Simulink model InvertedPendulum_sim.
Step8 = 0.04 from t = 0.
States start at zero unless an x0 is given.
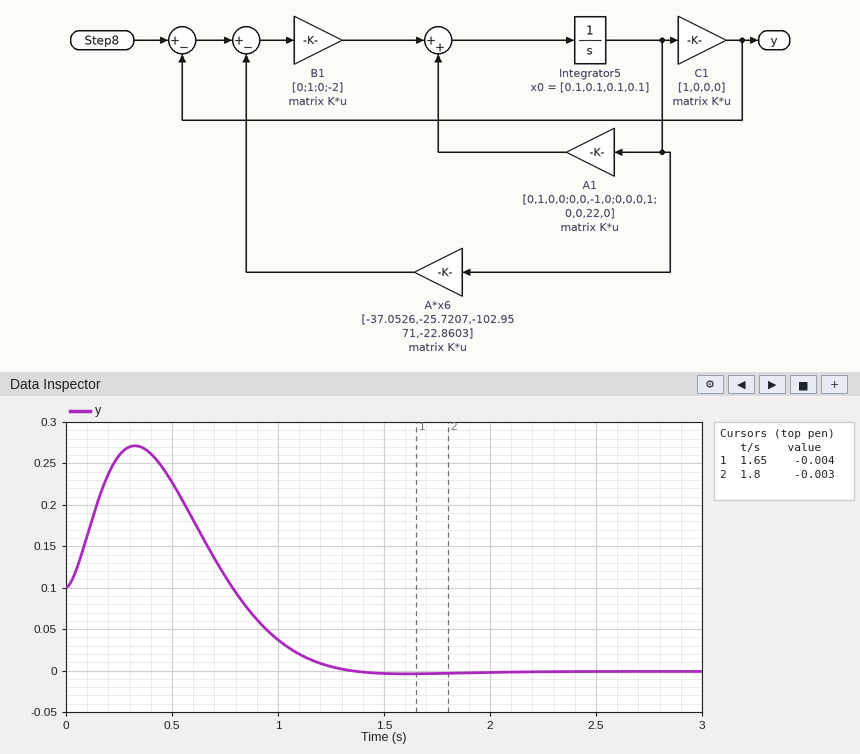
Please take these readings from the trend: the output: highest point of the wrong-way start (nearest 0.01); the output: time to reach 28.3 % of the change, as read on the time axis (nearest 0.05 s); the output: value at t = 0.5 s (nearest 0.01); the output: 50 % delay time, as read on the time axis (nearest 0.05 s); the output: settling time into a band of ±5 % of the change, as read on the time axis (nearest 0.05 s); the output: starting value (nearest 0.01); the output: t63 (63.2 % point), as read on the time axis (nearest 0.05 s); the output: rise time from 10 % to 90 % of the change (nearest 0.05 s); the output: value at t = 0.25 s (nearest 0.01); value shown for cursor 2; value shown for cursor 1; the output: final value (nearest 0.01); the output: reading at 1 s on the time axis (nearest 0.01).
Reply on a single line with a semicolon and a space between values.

0.27; 0.85 s; 0.23; 0.95 s; 1.25 s; 0.10; 1.00 s; 0.40 s; 0.26; -0.003; -0.004; 0.00; 0.04
